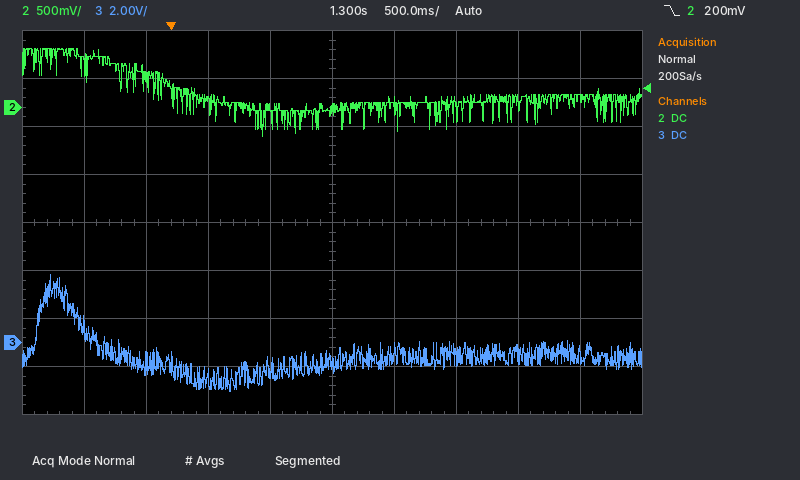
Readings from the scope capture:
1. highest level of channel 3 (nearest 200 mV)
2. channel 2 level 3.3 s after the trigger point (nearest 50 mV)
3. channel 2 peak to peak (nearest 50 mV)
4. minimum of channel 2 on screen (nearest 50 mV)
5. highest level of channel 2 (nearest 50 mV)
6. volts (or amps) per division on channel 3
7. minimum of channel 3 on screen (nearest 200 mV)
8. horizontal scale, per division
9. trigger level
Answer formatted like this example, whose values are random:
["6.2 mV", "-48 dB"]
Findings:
["2.8 V", "100 mV", "900 mV", "-300 mV", "600 mV", "2 V", "-2.0 V", "500 ms", "200 mV"]
